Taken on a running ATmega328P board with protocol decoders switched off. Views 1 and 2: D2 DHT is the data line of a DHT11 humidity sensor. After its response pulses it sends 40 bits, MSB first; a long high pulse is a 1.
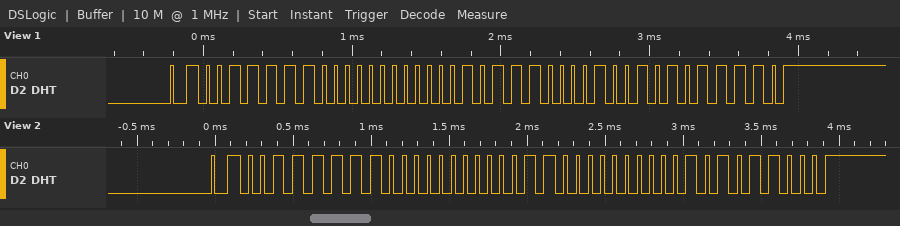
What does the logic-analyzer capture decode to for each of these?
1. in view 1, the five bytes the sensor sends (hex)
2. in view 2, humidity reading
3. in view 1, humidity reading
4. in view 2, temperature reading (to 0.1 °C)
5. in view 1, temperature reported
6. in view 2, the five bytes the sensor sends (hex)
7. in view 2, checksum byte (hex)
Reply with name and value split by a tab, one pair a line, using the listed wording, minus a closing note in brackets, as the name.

in view 1, the five bytes the sensor sends	3E 00 17 09 5E
in view 2, humidity reading	63 %
in view 1, humidity reading	62 %
in view 2, temperature reading	24.1 °C
in view 1, temperature reported	23.9 °C
in view 2, the five bytes the sensor sends	3F 00 18 01 58
in view 2, checksum byte	0x58
